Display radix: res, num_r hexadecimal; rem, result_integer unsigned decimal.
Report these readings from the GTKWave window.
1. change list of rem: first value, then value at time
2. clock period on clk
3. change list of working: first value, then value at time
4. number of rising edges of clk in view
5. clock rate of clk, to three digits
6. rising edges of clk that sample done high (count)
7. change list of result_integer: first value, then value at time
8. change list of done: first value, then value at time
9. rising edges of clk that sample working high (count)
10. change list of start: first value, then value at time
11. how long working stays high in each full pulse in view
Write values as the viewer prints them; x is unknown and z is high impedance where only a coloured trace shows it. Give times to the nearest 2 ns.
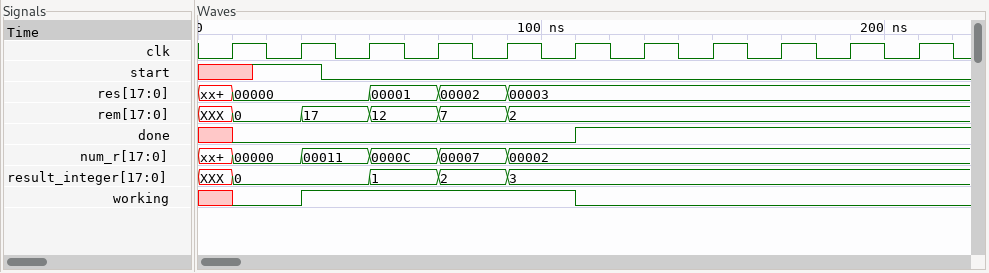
XXX, 0 at 10 ns, 17 at 30 ns, 12 at 50 ns, 7 at 70 ns, 2 at 90 ns
20 ns
x, 0 at 10 ns, 1 at 30 ns, 0 at 110 ns
11
50.0 MHz
5
XXX, 0 at 10 ns, 1 at 50 ns, 2 at 70 ns, 3 at 90 ns
x, 0 at 10 ns, 1 at 110 ns
4
x, 1 at 16 ns, 0 at 36 ns
80 ns
